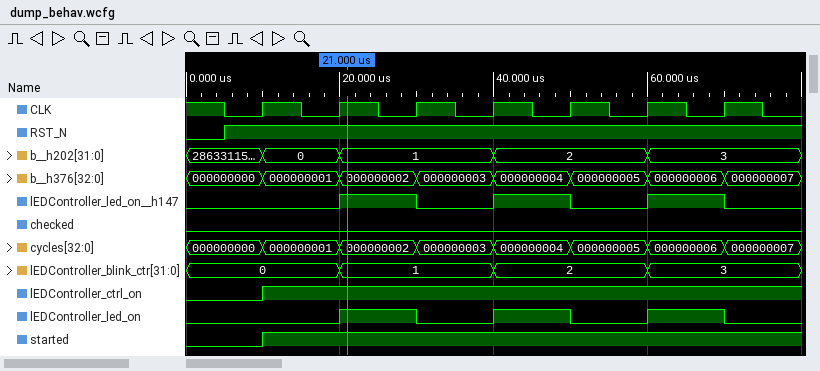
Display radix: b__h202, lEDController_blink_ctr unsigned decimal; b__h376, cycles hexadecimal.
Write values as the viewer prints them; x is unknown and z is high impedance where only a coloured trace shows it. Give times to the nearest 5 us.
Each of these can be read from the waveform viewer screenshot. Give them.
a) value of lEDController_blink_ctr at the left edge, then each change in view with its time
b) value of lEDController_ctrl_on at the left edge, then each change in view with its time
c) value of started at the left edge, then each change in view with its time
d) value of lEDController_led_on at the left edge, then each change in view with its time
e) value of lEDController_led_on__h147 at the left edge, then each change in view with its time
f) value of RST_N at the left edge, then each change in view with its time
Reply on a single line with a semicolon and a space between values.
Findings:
0, 1 at 20 us, 2 at 40 us, 3 at 60 us; 0, 1 at 10 us; 0, 1 at 10 us; 0, 1 at 20 us, 0 at 30 us, 1 at 40 us, 0 at 50 us, 1 at 60 us, 0 at 70 us; 0, 1 at 20 us, 0 at 30 us, 1 at 40 us, 0 at 50 us, 1 at 60 us, 0 at 70 us; 0, 1 at 5 us
